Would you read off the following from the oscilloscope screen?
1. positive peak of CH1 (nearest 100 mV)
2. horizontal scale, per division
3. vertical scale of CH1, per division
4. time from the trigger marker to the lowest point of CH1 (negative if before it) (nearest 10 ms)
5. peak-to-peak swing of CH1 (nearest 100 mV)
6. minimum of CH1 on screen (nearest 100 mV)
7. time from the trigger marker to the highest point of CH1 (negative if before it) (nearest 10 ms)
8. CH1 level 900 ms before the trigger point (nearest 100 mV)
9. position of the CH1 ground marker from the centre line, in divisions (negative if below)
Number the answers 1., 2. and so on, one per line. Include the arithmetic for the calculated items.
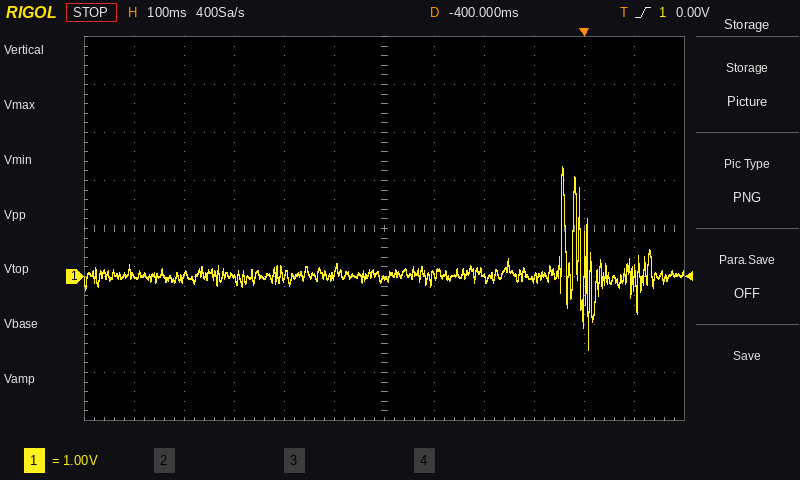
1. 2.3 V
2. 100 ms
3. 1 V
4. +10 ms
5. 2.3 V − (-1.5 V) = 3.8 V
6. -1.5 V
7. -40 ms
8. 0.0 V
9. -1.0 div
